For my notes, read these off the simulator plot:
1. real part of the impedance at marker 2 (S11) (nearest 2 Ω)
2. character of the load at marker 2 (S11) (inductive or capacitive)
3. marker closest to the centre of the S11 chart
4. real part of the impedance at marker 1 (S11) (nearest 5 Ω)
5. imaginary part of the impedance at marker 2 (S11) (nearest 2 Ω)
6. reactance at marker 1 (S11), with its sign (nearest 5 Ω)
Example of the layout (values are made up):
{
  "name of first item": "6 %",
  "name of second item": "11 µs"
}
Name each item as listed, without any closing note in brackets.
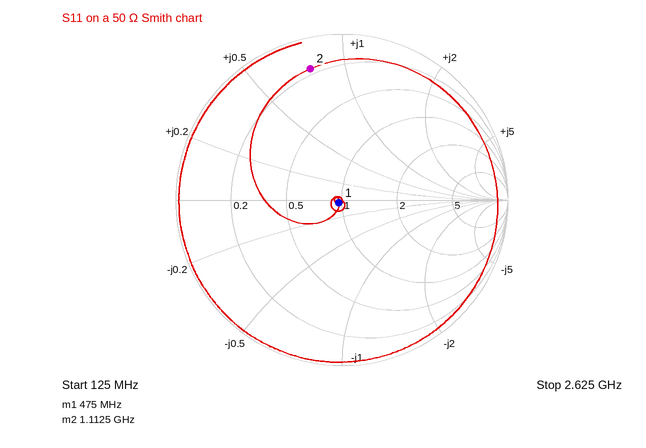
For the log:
{
  "real part of the impedance at marker 2 (S11)": "8 Ω",
  "character of the load at marker 2 (S11)": "inductive",
  "marker closest to the centre of the S11 chart": "marker 1",
  "real part of the impedance at marker 1 (S11)": "50 Ω",
  "imaginary part of the impedance at marker 2 (S11)": "+38 Ω",
  "reactance at marker 1 (S11), with its sign": "0 Ω"
}
